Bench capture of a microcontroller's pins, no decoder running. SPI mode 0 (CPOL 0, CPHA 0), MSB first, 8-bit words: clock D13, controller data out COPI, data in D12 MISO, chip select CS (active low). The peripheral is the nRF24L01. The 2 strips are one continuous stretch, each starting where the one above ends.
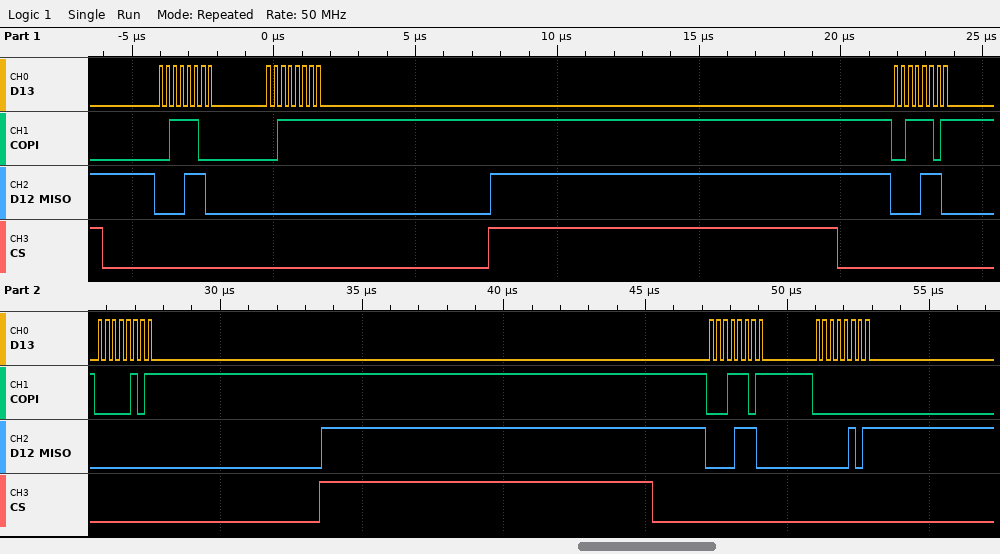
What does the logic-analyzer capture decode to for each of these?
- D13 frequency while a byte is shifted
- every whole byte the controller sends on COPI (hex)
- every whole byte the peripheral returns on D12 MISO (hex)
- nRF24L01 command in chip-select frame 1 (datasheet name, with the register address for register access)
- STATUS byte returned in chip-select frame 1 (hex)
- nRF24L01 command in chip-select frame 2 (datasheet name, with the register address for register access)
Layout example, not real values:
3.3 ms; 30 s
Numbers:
4 MHz; 3C 3F 3D 05 1D 00; 0E 00 0E 00 0E 05; W_REGISTER 0x1C; 0x0E; W_REGISTER 0x1D
